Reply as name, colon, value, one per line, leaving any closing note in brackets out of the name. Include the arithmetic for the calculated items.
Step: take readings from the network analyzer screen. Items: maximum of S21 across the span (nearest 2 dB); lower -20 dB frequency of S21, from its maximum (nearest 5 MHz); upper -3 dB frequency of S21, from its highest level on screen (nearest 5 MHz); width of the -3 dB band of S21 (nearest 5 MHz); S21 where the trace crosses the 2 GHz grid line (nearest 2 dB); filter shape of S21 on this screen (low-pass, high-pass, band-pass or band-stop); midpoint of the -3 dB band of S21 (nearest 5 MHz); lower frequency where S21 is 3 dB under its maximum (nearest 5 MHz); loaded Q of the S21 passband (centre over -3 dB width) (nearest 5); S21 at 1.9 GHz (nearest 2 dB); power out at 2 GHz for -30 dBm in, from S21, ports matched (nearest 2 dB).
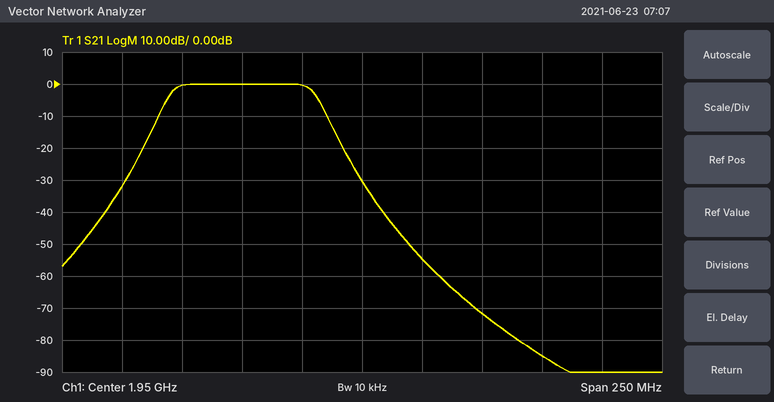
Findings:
maximum of S21 across the span: 0 dB
lower -20 dB frequency of S21, from its maximum: 1.860 GHz
upper -3 dB frequency of S21, from its highest level on screen: 1.930 GHz
width of the -3 dB band of S21: 1.930 GHz − 1.870 GHz = 60 MHz
S21 where the trace crosses the 2 GHz grid line: -72 dB
filter shape of S21 on this screen: band-pass
midpoint of the -3 dB band of S21: 1.900 GHz
lower frequency where S21 is 3 dB under its maximum: 1.870 GHz
loaded Q of the S21 passband (centre over -3 dB width): 1.9 GHz / 60 MHz ≈ 31.7, so 30 to the nearest 5
S21 at 1.9 GHz: 0 dB
power out at 2 GHz for -30 dBm in, from S21, ports matched: -30 dBm + (-72 dB) = -102 dBm
